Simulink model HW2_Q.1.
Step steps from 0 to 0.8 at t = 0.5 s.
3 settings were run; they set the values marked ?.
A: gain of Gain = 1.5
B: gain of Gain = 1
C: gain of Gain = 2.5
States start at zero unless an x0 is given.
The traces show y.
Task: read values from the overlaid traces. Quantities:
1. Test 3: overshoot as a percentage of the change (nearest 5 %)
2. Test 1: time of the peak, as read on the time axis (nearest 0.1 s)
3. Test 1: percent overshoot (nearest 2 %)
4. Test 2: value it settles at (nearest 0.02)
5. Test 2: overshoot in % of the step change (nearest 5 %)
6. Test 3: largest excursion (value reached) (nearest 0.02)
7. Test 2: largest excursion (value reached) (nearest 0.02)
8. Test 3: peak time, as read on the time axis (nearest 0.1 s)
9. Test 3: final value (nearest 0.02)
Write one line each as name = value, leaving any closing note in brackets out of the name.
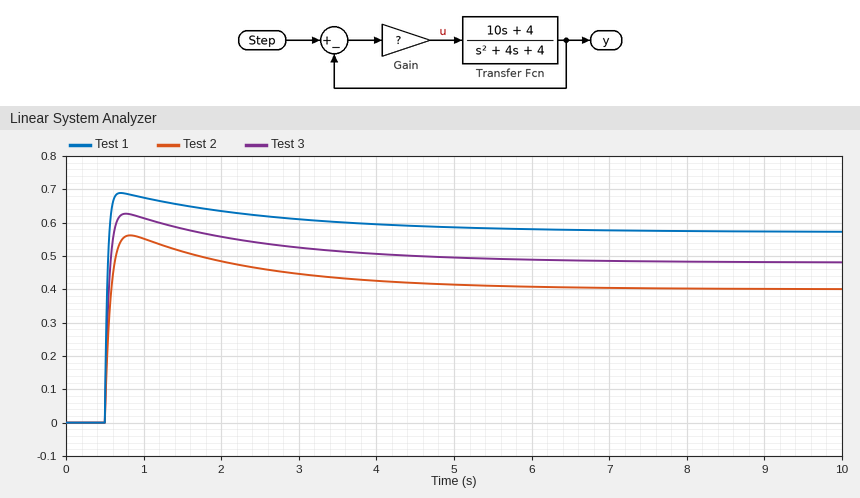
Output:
Test 3: overshoot as a percentage of the change = 30 %
Test 1: time of the peak, as read on the time axis = 0.7 s
Test 1: percent overshoot = 20 %
Test 2: value it settles at = 0.40
Test 2: overshoot in % of the step change = 40 %
Test 3: largest excursion (value reached) = 0.62
Test 2: largest excursion (value reached) = 0.56
Test 3: peak time, as read on the time axis = 0.8 s
Test 3: final value = 0.48
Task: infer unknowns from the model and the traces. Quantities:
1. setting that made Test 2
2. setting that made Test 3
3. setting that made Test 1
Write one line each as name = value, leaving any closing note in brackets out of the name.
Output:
setting that made Test 2 = B
setting that made Test 3 = A
setting that made Test 1 = C
